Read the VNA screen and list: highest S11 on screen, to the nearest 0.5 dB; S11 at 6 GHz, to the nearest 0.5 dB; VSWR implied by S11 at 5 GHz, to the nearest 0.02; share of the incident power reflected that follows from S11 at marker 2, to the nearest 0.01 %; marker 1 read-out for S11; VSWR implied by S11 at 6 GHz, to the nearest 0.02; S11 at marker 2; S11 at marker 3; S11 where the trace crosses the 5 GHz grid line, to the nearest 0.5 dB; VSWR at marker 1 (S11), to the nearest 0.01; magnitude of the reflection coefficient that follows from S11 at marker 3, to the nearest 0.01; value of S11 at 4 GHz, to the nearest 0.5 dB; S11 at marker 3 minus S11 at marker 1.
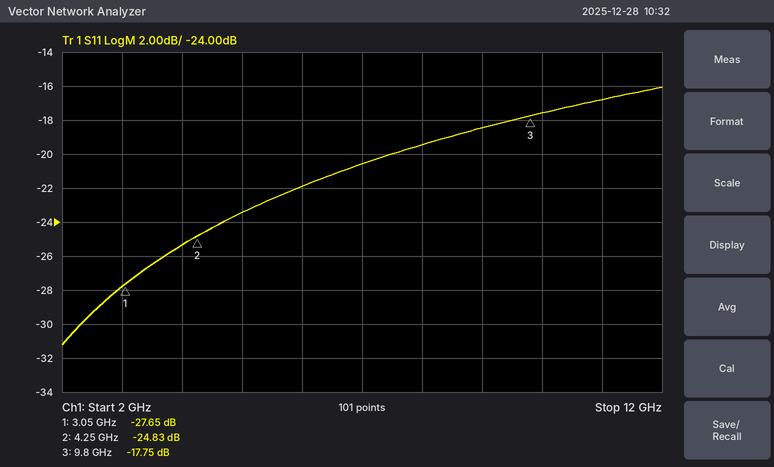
-16.0 dB
-22.0 dB
1.14
0.33 %
-27.65 dB
1.18
-24.83 dB
-17.75 dB
-23.5 dB
1.09
0.13
-25.5 dB
9.90 dB
